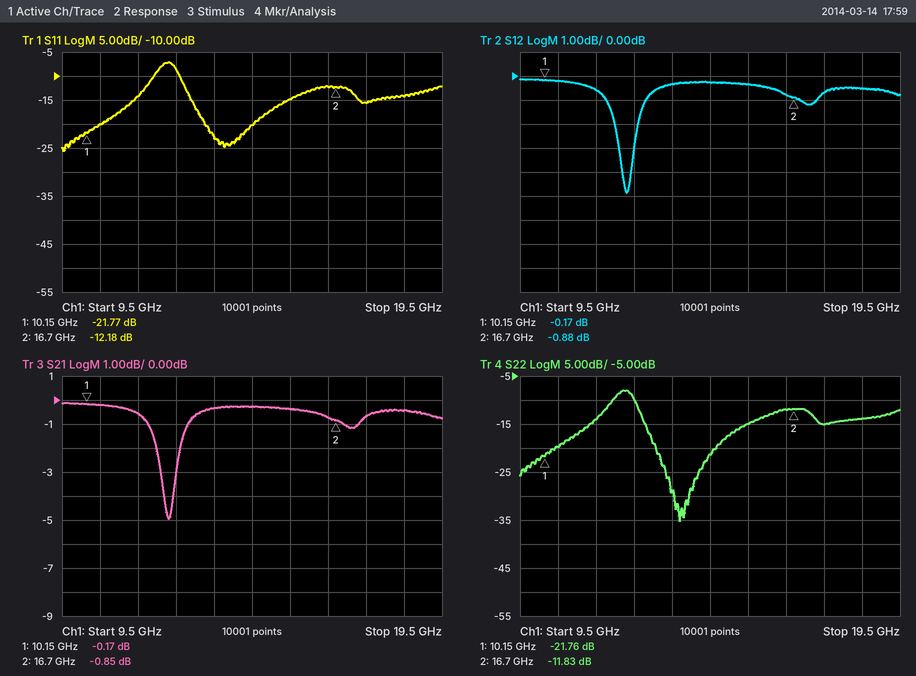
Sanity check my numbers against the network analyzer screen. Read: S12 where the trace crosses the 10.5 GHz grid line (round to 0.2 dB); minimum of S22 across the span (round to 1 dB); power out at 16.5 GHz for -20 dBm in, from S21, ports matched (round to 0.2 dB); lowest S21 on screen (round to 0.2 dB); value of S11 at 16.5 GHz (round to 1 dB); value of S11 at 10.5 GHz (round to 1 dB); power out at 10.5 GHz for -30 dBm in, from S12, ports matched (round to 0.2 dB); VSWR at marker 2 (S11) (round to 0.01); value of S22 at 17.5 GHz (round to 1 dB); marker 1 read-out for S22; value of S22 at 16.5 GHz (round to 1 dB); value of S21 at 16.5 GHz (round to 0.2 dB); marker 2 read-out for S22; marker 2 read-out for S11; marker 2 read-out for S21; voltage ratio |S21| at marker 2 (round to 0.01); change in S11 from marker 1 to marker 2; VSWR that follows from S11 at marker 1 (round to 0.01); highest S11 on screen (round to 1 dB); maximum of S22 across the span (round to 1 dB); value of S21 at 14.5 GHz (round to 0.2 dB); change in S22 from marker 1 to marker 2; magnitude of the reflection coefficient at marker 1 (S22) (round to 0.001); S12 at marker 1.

-0.2 dB
-35 dB
-20.8 dBm
-5.0 dB
-12 dB
-20 dB
-30.2 dBm
1.65
-15 dB
-21.76 dB
-12 dB
-0.8 dB
-11.83 dB
-12.18 dB
-0.85 dB
0.91
9.59 dB
1.18
-7 dB
-8 dB
-0.2 dB
9.93 dB
0.082
-0.17 dB
